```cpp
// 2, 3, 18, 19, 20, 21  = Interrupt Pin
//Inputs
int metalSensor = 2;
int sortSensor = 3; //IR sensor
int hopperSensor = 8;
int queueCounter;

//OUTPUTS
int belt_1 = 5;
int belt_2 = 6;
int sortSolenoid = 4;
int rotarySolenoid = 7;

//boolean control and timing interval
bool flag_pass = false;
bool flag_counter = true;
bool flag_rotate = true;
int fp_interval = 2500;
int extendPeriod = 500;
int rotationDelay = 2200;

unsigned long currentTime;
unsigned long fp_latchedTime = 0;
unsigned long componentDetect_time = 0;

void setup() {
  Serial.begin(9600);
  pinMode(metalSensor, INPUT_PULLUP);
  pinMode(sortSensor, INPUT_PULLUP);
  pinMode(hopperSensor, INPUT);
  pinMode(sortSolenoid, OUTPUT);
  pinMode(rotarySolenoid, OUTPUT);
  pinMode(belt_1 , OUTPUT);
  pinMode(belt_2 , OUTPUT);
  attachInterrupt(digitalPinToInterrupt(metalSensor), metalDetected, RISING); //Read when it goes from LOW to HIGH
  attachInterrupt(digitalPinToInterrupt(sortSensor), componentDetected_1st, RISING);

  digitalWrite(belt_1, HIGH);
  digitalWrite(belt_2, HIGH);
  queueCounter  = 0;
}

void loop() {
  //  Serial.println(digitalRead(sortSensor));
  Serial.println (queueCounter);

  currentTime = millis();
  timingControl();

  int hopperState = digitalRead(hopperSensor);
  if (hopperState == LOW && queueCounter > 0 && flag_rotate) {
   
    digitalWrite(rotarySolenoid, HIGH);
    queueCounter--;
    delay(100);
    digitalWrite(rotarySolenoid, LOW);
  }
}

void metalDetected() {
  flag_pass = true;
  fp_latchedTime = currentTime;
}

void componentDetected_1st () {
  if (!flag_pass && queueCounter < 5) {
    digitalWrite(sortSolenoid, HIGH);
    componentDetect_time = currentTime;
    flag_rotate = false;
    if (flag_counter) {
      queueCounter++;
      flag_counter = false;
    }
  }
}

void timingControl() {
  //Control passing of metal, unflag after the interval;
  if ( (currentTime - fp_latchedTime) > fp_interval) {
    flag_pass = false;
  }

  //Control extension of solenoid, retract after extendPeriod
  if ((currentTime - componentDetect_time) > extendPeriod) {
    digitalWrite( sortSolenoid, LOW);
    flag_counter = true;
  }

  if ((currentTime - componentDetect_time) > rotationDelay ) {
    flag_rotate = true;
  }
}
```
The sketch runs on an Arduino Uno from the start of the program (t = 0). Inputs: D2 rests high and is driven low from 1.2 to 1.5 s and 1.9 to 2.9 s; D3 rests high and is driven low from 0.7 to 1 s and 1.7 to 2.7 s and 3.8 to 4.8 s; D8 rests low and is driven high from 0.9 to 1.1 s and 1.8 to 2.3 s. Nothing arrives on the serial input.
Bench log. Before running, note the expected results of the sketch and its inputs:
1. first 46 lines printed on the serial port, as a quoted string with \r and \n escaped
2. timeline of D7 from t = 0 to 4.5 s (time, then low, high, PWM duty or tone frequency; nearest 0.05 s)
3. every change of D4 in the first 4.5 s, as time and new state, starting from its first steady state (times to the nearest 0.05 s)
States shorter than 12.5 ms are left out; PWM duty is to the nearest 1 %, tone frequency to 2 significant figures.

"0\r\n0\r\n0\r\n0\r\n0\r\n0\r\n0\r\n0\r\n0\r\n0\r\n0\r\n0\r\n0\r\n0\r\n0\r\n0\r\n0\r\n0\r\n0\r\n0\r\n0\r\n0\r\n0\r\n0\r\n0\r\n0\r\n0\r\n0\r\n0\r\n0\r\n0\r\n0\r\n0\r\n0\r\n0\r\n0\r\n0\r\n0\r\n0\r\n0\r\n0\r\n0\r\n0\r\n0\r\n0\r\n0\r\n"
0 s low; 3.2 s high; 3.3 s low
0 s low; 1 s high; 1.5 s low
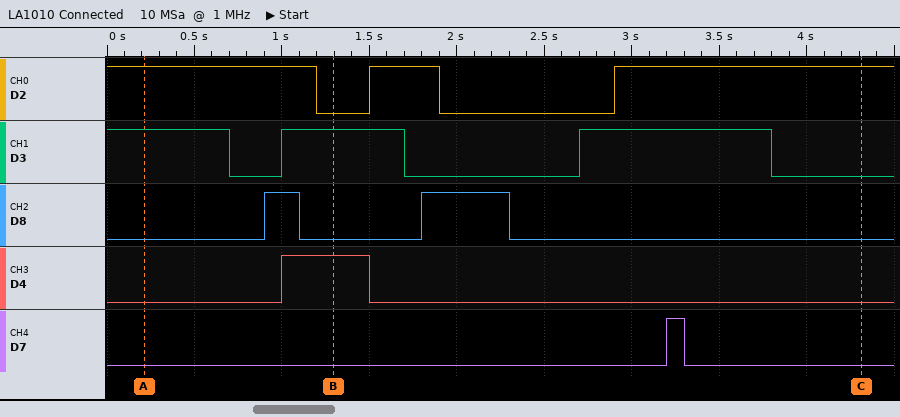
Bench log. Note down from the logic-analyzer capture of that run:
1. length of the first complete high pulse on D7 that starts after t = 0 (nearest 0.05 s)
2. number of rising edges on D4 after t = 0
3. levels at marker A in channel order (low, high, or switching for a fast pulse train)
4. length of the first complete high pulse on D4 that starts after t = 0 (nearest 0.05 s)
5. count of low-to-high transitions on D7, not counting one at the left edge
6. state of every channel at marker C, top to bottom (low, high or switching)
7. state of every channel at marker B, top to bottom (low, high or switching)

0.10 s
1
D2 high, D3 high, D8 low, D4 low, D7 low
0.50 s
1
D2 high, D3 low, D8 low, D4 low, D7 low
D2 low, D3 high, D8 low, D4 high, D7 low
